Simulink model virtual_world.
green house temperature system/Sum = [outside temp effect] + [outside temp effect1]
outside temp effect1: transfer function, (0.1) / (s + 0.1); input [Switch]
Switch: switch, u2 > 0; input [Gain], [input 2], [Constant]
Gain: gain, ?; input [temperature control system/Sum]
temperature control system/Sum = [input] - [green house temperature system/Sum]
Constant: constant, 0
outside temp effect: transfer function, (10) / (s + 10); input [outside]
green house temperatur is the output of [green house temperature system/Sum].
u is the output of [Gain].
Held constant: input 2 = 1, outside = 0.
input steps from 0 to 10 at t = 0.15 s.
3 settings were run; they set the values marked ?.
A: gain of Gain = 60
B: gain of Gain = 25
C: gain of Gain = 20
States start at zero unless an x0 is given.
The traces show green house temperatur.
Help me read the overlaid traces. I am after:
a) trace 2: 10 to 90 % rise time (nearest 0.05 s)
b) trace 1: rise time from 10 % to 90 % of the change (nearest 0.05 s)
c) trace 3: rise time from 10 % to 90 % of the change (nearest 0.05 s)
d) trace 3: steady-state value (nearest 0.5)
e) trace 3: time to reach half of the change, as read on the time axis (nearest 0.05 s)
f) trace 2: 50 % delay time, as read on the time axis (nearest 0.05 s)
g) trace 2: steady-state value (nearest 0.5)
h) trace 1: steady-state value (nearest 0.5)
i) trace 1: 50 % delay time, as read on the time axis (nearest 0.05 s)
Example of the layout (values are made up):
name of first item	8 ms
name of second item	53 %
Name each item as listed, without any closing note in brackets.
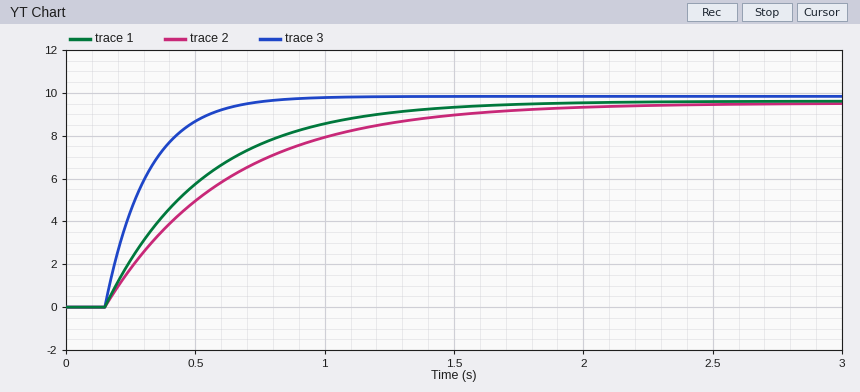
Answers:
trace 2: 10 to 90 % rise time	1.05 s
trace 1: rise time from 10 % to 90 % of the change	0.85 s
trace 3: rise time from 10 % to 90 % of the change	0.35 s
trace 3: steady-state value	10.0
trace 3: time to reach half of the change, as read on the time axis	0.25 s
trace 2: 50 % delay time, as read on the time axis	0.50 s
trace 2: steady-state value	9.5
trace 1: steady-state value	9.5
trace 1: 50 % delay time, as read on the time axis	0.40 s
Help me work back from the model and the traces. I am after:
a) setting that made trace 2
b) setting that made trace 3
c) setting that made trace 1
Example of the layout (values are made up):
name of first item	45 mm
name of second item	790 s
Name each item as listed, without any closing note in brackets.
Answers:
setting that made trace 2	C
setting that made trace 3	A
setting that made trace 1	B
